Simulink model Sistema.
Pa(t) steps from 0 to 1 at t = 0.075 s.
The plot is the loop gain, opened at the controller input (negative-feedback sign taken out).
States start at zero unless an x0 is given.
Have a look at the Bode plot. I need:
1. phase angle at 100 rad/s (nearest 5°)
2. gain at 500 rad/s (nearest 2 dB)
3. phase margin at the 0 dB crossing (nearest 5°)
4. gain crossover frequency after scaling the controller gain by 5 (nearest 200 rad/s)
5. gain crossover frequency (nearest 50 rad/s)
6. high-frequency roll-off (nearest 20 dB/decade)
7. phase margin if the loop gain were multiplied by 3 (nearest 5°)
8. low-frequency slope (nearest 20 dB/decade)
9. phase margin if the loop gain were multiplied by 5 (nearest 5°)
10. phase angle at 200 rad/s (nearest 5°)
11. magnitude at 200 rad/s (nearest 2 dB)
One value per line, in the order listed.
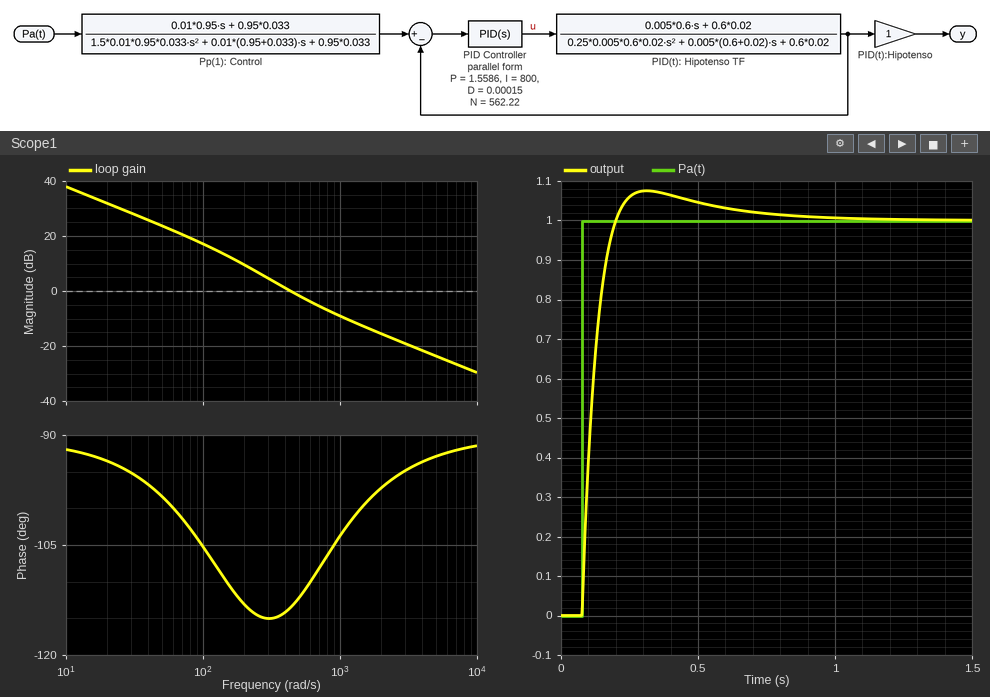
-105°
-2 dB
65°
1600 rad/s
450 rad/s
-20 dB/decade
75°
-20 dB/decade
80°
-115°
10 dB
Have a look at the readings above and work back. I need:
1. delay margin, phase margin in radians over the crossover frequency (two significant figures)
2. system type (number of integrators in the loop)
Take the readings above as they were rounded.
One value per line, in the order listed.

0.0025 s
1
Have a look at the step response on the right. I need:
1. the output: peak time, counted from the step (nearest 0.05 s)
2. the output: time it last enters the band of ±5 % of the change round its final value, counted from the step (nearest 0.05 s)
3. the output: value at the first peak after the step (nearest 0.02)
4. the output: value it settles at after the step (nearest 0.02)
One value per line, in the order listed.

0.25 s
0.40 s
1.08
1.00
